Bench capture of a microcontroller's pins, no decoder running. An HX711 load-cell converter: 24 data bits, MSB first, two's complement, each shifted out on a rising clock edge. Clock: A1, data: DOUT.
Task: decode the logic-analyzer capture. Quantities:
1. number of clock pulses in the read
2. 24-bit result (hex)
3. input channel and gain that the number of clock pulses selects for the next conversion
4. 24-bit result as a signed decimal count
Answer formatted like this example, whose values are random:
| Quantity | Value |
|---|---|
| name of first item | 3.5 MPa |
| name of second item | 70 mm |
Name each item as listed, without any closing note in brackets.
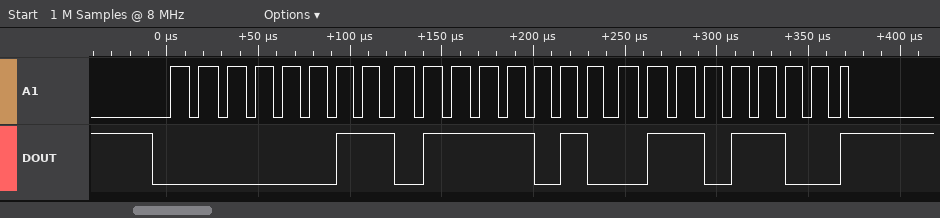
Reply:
| Quantity | Value |
|---|---|
| number of clock pulses in the read | 25 |
| 24-bit result | 0x037A6C |
| input channel and gain that the number of clock pulses selects for the next conversion | channel A, gain 128 |
| 24-bit result as a signed decimal count | 227948 |
